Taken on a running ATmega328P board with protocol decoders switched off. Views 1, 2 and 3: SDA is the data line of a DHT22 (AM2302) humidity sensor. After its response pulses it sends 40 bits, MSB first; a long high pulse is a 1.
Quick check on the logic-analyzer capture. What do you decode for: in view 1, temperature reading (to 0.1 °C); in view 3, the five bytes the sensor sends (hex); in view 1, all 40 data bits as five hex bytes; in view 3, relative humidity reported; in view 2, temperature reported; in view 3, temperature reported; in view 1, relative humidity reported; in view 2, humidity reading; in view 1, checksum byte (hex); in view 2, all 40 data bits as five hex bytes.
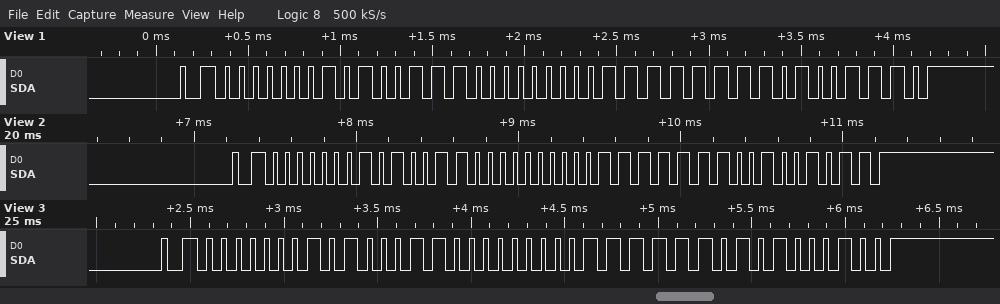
25.5 °C
01 46 00 FD 44
01 4E 00 FF 4E
32.6 %
25.4 °C
25.3 °C
33.4 %
33.2 %
0x4E
01 4C 00 FE 4B
